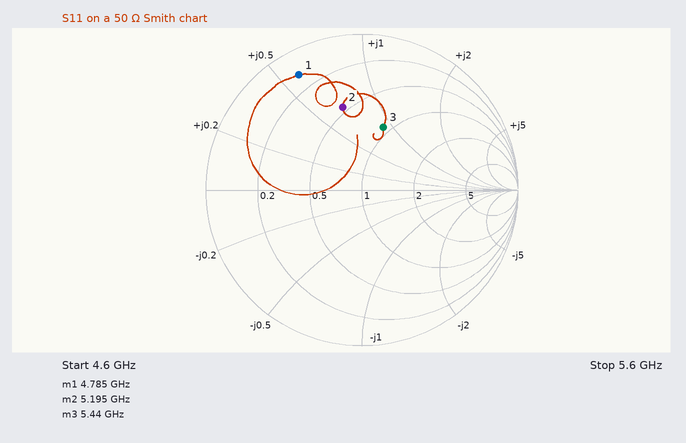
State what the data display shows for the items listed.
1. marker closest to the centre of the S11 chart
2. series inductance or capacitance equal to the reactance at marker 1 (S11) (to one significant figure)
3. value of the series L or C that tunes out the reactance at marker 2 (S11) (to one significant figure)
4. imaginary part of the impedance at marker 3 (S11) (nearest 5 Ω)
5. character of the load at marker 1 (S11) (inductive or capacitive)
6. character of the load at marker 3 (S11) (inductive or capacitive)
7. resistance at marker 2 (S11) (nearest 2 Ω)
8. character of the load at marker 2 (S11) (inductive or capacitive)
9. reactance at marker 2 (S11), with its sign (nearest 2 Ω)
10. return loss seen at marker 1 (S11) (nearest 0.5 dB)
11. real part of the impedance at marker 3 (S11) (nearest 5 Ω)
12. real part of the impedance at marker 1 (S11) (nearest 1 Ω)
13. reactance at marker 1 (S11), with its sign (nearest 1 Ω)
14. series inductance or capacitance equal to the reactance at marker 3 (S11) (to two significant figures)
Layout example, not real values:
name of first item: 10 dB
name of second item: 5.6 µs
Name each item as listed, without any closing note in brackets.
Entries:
marker closest to the centre of the S11 chart: marker 3
series inductance or capacitance equal to the reactance at marker 1 (S11): 1.0 nH
value of the series L or C that tunes out the reactance at marker 2 (S11): 900 fF
imaginary part of the impedance at marker 3 (S11): +45 Ω
character of the load at marker 1 (S11): inductive
character of the load at marker 3 (S11): inductive
resistance at marker 2 (S11): 22 Ω
character of the load at marker 2 (S11): inductive
reactance at marker 2 (S11), with its sign: +34 Ω
return loss seen at marker 1 (S11): 1.5 dB
real part of the impedance at marker 3 (S11): 45 Ω
real part of the impedance at marker 1 (S11): 6 Ω
reactance at marker 1 (S11), with its sign: +29 Ω
series inductance or capacitance equal to the reactance at marker 3 (S11): 1.3 nH
